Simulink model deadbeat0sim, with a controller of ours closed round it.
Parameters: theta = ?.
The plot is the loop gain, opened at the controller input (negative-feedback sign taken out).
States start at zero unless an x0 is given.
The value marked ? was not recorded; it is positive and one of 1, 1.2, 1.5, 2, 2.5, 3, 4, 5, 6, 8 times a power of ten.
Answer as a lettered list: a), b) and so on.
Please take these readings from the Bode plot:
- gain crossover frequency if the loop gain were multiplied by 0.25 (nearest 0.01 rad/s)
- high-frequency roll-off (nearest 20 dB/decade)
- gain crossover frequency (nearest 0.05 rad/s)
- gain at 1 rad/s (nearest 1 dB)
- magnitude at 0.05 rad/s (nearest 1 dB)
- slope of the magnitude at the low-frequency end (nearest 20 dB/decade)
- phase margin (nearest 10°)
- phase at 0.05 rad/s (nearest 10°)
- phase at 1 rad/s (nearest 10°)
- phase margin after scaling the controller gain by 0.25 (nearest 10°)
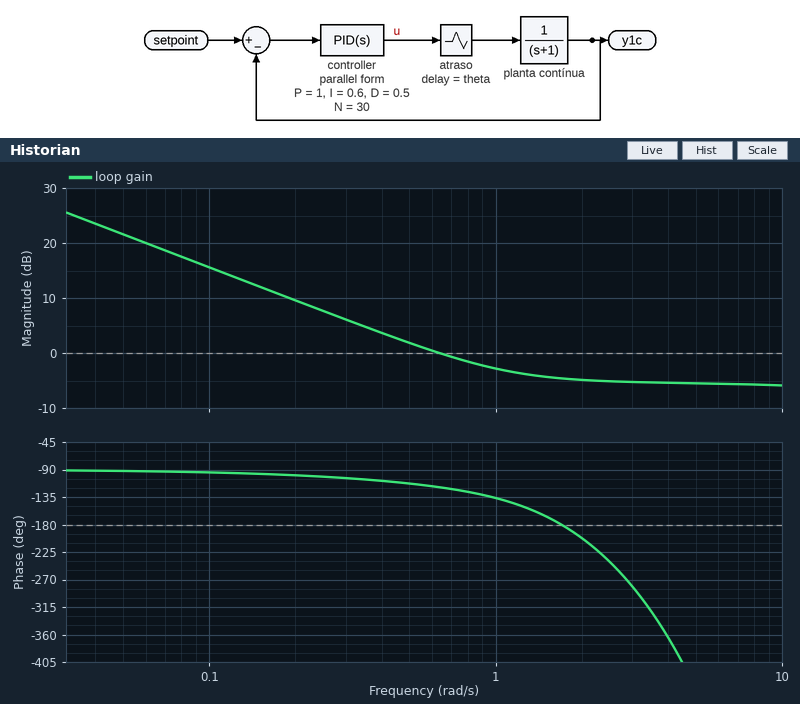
a) 0.15 rad/s
b) 0 dB/decade
c) 0.65 rad/s
d) -3 dB
e) 22 dB
f) -20 dB/decade
g) 60°
h) -90°
i) -140°
j) 80°
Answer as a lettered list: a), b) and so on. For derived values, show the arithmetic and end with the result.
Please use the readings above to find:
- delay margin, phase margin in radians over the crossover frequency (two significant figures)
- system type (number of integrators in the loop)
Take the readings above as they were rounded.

a) 60 × π / 180 / 0.65 = 1.6 s
b) 1
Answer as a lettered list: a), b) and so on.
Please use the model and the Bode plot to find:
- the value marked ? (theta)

a) 1.5
